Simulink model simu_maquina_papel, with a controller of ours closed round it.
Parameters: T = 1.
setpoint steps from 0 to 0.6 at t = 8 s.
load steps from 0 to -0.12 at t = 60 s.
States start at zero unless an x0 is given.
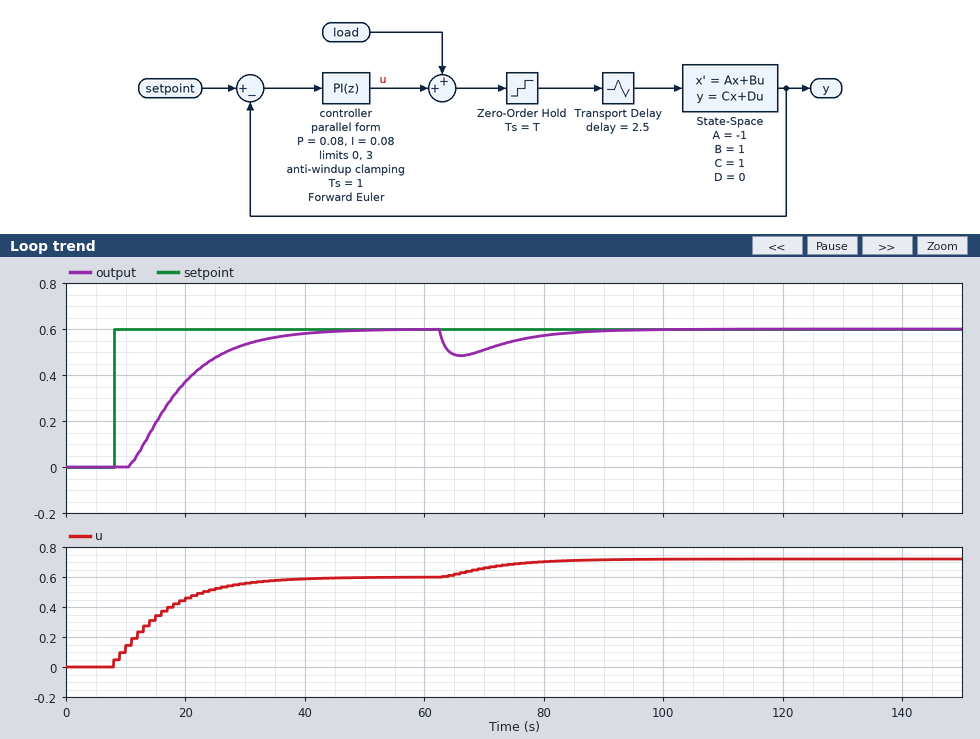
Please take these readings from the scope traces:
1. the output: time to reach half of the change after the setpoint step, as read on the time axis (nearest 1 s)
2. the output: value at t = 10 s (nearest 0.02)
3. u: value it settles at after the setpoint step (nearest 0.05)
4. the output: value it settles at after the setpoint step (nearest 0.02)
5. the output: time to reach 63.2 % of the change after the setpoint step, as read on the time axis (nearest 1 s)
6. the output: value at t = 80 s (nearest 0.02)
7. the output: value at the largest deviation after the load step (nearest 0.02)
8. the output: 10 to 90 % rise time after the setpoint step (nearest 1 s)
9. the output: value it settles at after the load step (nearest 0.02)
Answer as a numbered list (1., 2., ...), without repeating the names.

1. 18 s
2. 0.00
3. 0.60
4. 0.60
5. 20 s
6. 0.58
7. 0.48
8. 19 s
9. 0.60
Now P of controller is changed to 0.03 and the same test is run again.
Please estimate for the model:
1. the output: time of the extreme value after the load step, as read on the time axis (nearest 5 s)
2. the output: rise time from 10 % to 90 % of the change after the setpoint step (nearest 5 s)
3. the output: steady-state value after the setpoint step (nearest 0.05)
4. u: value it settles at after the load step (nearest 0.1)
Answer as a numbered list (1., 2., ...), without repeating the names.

1. 65 s
2. 15 s
3. 0.60
4. 0.7
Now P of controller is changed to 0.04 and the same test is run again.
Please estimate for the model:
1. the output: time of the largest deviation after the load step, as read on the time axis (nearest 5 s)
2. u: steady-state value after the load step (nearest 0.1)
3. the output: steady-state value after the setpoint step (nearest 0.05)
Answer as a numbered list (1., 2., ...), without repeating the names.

1. 65 s
2. 0.7
3. 0.60
